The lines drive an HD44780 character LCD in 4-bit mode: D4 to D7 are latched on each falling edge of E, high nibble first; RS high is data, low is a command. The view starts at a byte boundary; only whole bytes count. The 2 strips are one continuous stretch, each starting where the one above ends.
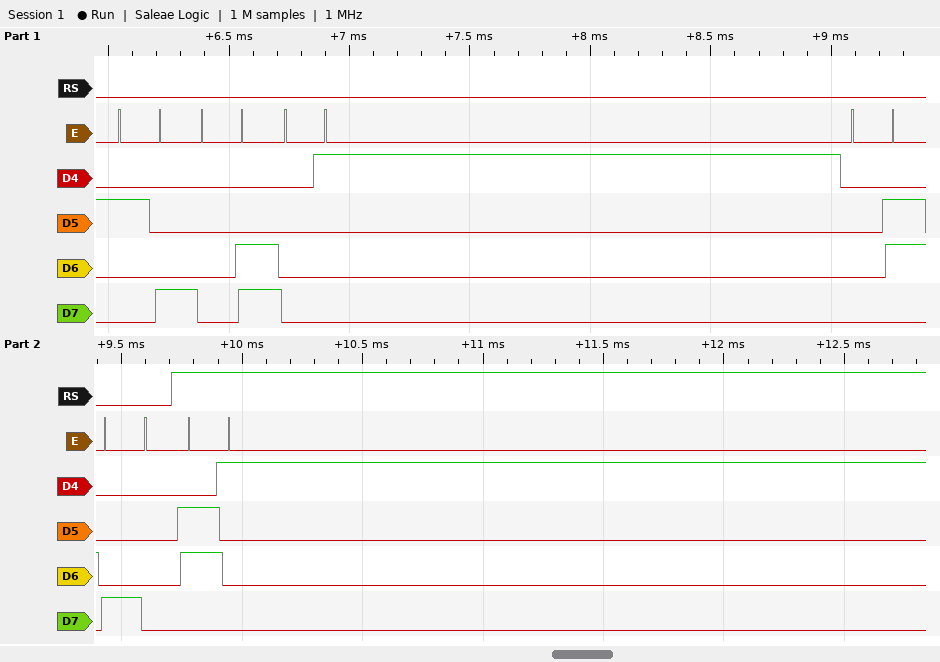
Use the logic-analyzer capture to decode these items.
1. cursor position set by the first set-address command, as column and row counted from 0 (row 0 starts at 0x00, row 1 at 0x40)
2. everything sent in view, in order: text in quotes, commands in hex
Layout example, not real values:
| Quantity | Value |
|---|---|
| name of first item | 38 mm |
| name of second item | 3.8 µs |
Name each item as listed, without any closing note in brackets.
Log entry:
| Quantity | Value |
|---|---|
| cursor position set by the first set-address command, as column and row counted from 0 | column 0, row 0 |
| everything sent in view, in order: text in quotes, commands in hex | 0x28 0x0C 0x01 0x06 0x80 "a" |
